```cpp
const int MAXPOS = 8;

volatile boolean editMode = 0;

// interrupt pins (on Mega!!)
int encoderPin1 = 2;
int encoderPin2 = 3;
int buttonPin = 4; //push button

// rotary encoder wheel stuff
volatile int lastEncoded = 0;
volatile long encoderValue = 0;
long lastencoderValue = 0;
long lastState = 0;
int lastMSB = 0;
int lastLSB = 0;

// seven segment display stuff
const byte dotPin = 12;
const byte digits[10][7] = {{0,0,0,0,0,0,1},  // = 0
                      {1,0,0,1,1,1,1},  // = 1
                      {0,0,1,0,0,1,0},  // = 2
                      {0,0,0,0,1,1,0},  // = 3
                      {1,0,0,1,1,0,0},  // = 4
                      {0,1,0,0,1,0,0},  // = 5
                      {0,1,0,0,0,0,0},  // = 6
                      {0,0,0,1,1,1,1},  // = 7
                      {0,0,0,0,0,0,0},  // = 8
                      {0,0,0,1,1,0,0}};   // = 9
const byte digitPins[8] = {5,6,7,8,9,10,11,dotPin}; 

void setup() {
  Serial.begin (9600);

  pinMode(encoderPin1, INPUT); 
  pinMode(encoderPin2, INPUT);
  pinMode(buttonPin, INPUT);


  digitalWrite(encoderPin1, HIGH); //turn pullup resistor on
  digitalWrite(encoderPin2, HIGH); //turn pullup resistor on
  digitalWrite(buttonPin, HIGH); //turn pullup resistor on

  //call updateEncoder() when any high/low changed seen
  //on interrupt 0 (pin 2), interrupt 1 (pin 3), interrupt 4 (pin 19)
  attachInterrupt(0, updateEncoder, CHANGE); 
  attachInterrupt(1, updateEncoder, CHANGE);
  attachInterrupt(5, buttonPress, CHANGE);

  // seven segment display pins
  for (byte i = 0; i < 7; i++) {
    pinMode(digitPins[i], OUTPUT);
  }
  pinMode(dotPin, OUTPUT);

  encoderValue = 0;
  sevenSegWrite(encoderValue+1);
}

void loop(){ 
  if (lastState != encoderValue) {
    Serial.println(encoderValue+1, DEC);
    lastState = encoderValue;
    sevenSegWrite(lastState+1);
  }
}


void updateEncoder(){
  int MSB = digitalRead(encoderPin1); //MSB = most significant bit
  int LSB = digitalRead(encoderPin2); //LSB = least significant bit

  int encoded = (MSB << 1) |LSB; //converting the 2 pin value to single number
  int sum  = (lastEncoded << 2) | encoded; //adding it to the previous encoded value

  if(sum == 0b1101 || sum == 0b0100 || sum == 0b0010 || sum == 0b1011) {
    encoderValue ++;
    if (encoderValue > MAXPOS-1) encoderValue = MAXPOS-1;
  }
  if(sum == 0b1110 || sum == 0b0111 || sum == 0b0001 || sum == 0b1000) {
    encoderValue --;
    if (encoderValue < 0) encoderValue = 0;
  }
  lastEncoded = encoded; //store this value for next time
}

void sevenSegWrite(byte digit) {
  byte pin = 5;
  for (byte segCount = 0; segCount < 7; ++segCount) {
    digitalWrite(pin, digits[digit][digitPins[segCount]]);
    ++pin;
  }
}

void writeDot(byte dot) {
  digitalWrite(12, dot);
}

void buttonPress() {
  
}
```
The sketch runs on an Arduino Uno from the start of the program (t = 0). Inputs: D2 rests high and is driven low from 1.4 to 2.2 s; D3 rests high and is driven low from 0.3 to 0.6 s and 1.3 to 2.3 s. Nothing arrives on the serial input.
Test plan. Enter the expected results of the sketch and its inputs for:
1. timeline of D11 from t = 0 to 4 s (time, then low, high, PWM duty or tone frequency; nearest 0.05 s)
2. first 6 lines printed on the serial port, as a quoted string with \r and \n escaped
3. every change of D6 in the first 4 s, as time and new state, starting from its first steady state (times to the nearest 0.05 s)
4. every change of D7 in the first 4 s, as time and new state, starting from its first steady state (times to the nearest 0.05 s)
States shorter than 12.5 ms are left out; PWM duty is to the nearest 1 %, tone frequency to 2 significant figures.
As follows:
0 s low; 0.3 s high; 1.4 s low; 2.2 s high
"2\r\n3\r\n2\r\n1\r\n2\r\n3\r\n"
0 s high; 0.3 s low; 1.4 s high; 2.2 s low
0 s low; 0.6 s high; 1.3 s low; 2.3 s high
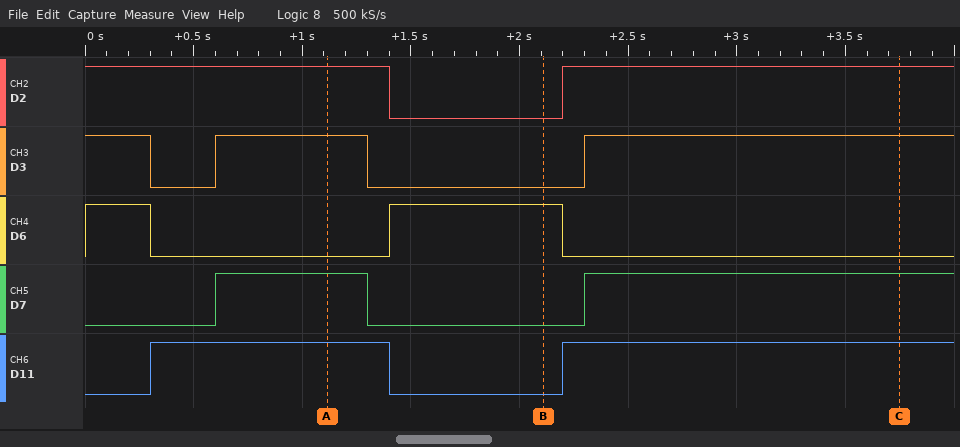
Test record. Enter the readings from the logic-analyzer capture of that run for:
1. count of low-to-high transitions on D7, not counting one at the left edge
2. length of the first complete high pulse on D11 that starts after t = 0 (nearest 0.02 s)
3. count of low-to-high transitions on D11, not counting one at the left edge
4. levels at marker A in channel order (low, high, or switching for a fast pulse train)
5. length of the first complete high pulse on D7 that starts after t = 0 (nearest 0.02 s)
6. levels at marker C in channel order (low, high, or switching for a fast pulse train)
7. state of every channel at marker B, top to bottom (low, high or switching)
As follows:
2
1.10 s
2
D2 high, D3 high, D6 low, D7 high, D11 high
0.70 s
D2 high, D3 high, D6 low, D7 high, D11 high
D2 low, D3 low, D6 high, D7 low, D11 low
